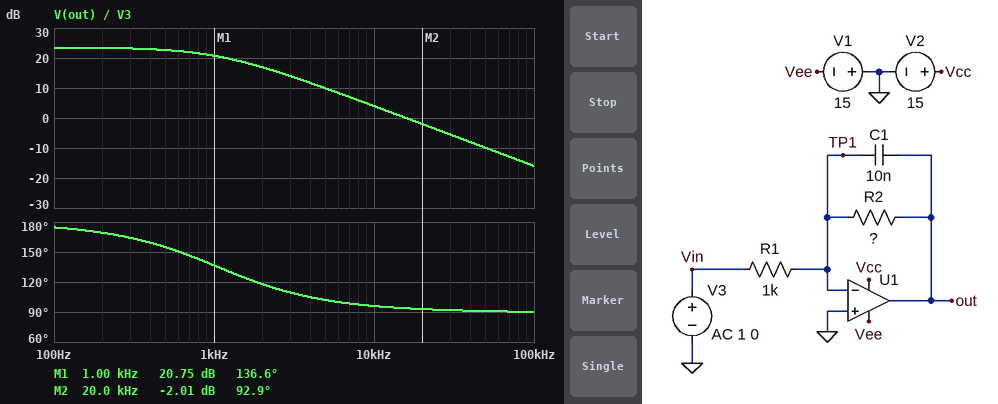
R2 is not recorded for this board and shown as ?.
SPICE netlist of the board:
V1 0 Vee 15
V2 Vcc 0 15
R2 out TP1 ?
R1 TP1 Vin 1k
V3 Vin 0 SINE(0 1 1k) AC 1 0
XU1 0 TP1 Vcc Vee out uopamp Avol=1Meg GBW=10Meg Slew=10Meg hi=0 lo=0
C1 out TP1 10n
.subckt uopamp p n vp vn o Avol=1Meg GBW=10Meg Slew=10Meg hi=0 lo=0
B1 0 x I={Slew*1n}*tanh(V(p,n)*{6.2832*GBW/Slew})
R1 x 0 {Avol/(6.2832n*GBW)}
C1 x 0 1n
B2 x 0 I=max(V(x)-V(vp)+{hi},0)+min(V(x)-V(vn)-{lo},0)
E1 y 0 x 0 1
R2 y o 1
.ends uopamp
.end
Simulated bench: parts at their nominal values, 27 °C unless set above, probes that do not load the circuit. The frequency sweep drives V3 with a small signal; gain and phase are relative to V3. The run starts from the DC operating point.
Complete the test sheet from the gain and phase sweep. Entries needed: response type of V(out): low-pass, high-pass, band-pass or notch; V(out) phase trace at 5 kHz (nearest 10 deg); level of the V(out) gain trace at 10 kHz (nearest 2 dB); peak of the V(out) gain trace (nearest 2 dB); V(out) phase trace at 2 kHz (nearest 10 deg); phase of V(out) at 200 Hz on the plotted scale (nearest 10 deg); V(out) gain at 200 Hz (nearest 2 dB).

low-pass
100 deg
4 dB
24 dB
120 deg
170 deg
24 dB
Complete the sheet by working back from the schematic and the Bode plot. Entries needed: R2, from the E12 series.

15 kΩ
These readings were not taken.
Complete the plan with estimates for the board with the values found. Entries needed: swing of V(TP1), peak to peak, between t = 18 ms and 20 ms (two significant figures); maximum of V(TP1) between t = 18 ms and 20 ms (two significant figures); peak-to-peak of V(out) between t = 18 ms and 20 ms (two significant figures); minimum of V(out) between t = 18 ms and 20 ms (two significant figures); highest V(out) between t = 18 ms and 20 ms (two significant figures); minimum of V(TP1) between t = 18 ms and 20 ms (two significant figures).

2.2 mV
1.1 mV
22 V
-11 V
11 V
-1.1 mV
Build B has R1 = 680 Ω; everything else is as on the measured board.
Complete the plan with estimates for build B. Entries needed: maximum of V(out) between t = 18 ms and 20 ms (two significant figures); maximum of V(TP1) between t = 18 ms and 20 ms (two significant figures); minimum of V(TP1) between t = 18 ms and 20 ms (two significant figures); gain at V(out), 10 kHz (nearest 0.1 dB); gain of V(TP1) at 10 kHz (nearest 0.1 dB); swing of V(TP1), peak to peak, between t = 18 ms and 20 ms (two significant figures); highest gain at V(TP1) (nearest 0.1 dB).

15 V
190 mV
-190 mV
7.3 dB
-52.7 dB
380 mV
-52.6 dB
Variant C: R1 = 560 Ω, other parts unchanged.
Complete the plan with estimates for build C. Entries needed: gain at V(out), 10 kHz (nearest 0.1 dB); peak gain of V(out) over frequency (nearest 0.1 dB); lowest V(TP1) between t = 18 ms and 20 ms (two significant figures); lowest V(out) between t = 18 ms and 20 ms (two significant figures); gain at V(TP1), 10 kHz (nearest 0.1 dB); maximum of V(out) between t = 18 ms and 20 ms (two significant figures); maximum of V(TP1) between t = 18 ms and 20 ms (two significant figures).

9.0 dB
28.6 dB
-410 mV
-15 V
-51.0 dB
15 V
410 mV
